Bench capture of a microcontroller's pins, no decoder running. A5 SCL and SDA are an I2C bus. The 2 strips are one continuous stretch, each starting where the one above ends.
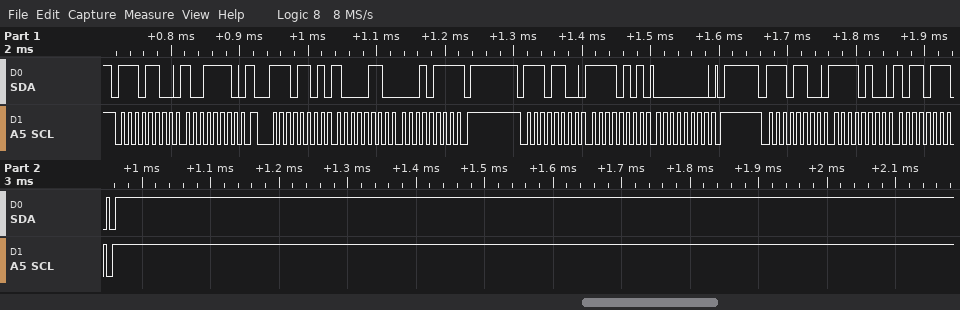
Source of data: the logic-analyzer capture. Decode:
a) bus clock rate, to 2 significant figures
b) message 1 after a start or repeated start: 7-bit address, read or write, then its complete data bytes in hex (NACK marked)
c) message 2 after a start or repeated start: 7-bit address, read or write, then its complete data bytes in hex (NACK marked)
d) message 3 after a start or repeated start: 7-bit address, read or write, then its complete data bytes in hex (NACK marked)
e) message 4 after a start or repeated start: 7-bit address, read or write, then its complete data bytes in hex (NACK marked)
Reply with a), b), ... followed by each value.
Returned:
a) 100 kHz
b) 0x76 write: 9E
c) 0x76 read: 86 17 NACK
d) 0x76 write: F5 00
e) 0x76 write: F4 B7
